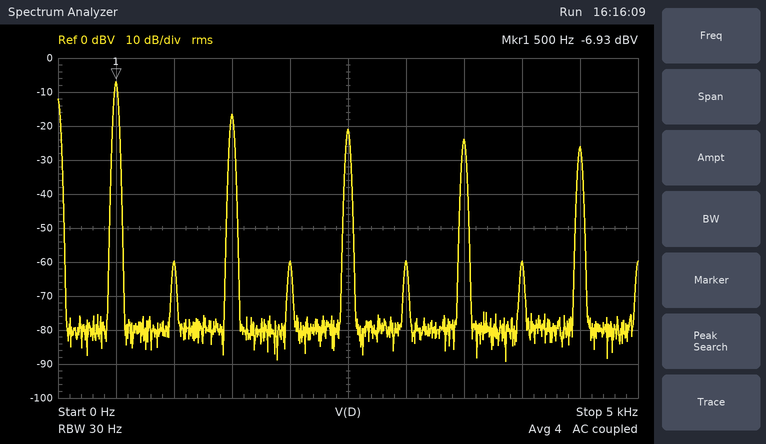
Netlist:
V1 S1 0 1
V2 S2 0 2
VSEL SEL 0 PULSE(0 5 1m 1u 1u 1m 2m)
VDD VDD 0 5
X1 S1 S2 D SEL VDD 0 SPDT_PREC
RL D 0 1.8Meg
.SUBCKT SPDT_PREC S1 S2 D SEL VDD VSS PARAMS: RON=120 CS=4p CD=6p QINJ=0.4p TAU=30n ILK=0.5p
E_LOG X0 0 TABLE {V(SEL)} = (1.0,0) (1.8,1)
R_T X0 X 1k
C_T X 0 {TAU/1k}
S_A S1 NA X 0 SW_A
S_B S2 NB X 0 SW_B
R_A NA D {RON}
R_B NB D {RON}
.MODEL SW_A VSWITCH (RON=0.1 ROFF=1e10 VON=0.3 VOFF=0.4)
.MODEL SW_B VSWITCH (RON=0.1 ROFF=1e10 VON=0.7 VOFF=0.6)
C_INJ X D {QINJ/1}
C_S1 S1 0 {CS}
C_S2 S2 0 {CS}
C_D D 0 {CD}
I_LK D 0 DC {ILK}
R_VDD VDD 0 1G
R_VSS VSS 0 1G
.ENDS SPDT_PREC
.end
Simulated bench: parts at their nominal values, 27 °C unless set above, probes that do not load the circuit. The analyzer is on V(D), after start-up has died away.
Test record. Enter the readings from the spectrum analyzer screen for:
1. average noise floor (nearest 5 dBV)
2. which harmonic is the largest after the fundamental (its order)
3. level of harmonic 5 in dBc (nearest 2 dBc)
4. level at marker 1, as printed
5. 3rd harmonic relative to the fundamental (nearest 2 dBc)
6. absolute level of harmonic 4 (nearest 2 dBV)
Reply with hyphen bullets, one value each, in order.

- -80 dBV
- 3
- -14 dBc
- -6.93 dBV
- -10 dBc
- -60 dBV
